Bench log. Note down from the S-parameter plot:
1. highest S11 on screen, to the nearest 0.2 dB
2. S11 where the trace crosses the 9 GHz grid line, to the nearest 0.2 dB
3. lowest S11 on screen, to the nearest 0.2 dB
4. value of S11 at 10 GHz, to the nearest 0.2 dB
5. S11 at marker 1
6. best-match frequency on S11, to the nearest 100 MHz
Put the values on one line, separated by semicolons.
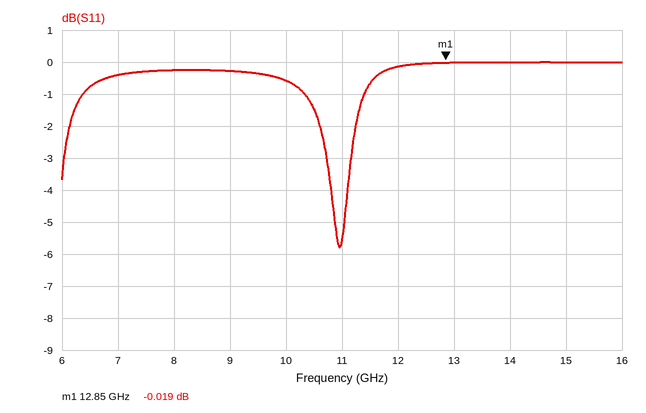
0.0 dB; -0.2 dB; -5.8 dB; -0.6 dB; -0.019 dB; 11.0 GHz
